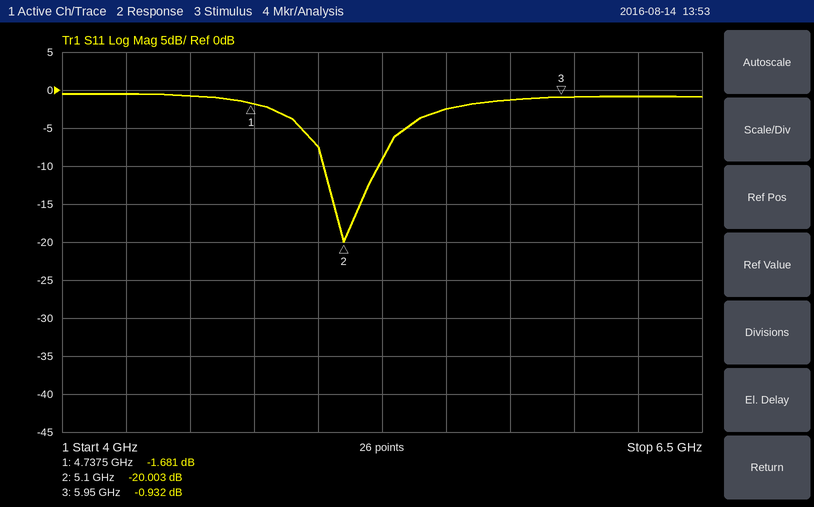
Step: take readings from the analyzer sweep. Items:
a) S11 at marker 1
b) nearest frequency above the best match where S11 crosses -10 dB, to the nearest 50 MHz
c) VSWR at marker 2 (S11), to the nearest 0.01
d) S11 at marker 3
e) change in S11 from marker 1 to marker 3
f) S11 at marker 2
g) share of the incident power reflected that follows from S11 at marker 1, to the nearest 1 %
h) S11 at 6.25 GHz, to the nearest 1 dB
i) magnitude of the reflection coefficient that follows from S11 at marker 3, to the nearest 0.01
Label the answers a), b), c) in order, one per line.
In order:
a) -1.681 dB
b) 5.25 GHz
c) 1.22
d) -0.932 dB
e) 0.749 dB
f) -20.003 dB
g) 68 %
h) -1 dB
i) 0.90
